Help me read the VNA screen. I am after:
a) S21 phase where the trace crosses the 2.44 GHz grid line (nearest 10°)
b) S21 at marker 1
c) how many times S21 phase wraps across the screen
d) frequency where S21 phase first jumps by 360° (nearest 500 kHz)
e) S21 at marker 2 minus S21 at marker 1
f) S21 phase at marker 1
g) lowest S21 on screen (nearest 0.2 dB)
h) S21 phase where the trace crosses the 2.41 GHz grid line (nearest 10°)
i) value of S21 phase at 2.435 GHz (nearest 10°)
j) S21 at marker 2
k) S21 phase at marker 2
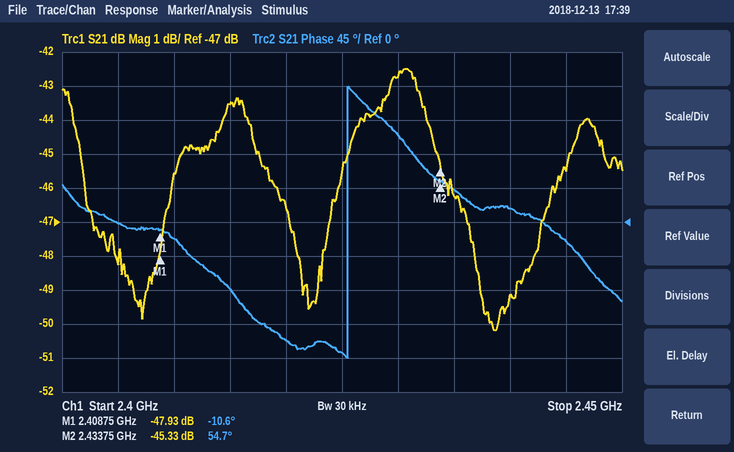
20°
-47.93 dB
1
2.4255 GHz
2.60 dB
-10.6°
-50.2 dB
-20°
40°
-45.33 dB
54.7°
